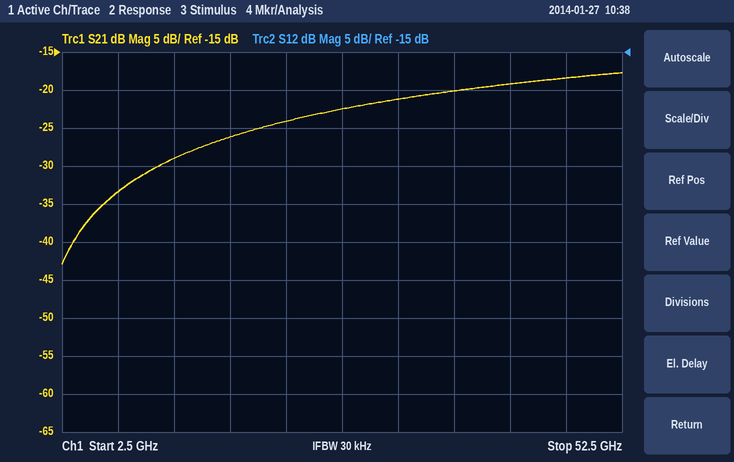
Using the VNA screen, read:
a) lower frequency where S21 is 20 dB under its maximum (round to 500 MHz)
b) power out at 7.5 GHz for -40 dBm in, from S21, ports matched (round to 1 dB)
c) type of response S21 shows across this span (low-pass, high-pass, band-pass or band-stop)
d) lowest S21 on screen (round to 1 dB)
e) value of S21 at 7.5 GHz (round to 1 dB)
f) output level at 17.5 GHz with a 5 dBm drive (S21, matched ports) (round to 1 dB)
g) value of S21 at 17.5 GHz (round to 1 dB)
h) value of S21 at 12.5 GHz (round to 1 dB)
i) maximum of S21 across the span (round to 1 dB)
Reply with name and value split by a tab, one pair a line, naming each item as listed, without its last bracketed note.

lower frequency where S21 is 20 dB under its maximum	4.5 GHz
power out at 7.5 GHz for -40 dBm in, from S21, ports matched	-73 dBm
type of response S21 shows across this span	high-pass
lowest S21 on screen	-43 dB
value of S21 at 7.5 GHz	-33 dB
output level at 17.5 GHz with a 5 dBm drive (S21, matched ports)	-21 dBm
value of S21 at 17.5 GHz	-26 dB
value of S21 at 12.5 GHz	-29 dB
maximum of S21 across the span	-18 dB
